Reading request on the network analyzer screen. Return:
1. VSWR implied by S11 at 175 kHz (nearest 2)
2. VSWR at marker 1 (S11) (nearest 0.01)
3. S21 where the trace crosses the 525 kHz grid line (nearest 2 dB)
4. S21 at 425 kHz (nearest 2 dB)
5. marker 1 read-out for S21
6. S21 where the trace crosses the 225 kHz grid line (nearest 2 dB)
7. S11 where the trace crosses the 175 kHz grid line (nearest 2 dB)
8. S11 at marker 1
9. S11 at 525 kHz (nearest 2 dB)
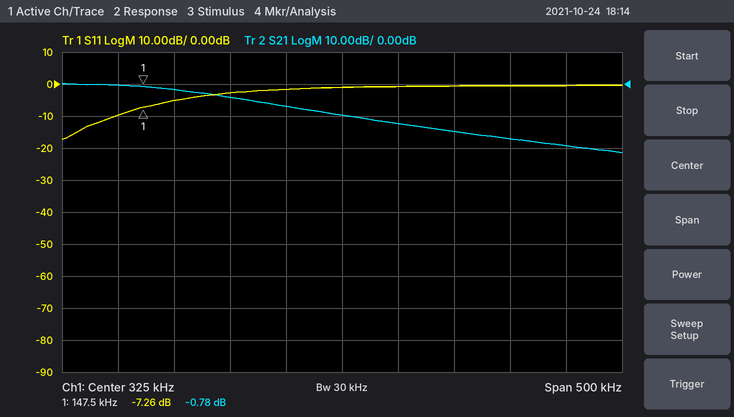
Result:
4
2.53
-20 dB
-14 dB
-0.78 dB
-4 dB
-6 dB
-7.26 dB
0 dB
